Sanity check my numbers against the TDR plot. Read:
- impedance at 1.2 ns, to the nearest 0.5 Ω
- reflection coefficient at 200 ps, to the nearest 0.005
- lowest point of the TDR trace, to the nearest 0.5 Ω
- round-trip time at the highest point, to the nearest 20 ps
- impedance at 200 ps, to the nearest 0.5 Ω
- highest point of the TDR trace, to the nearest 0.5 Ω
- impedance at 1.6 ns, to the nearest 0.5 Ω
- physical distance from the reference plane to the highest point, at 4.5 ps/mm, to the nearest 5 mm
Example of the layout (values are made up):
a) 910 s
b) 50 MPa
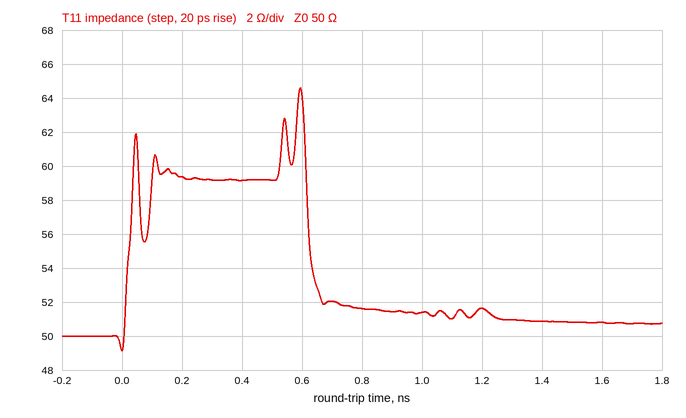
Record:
a) 51.5 Ω
b) +0.085
c) 49.0 Ω
d) 600 ps
e) 59.5 Ω
f) 64.5 Ω
g) 51.0 Ω
h) 65 mm
